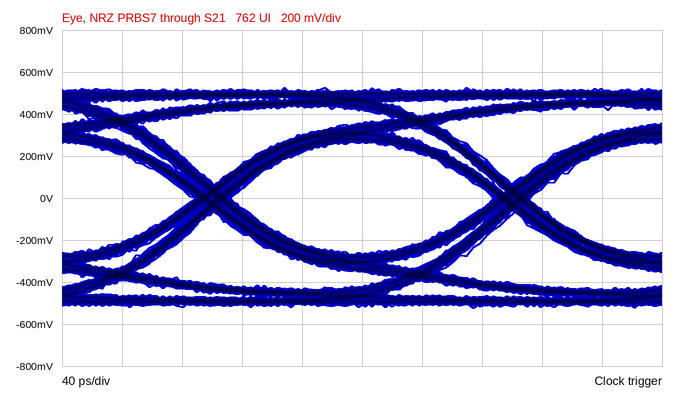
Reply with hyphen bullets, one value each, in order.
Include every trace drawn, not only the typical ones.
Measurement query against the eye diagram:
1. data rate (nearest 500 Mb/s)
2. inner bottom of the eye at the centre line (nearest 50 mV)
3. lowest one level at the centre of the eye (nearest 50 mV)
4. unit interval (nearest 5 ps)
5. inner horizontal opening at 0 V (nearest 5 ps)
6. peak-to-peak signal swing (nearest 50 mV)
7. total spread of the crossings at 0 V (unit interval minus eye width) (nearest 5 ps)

- 5.0 Gb/s
- -250 mV
- 250 mV
- 200 ps
- 175 ps
- 1.05 V
- 25 ps
